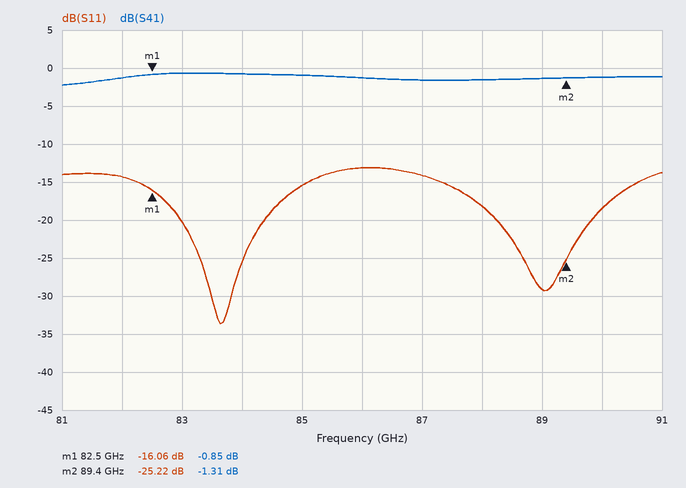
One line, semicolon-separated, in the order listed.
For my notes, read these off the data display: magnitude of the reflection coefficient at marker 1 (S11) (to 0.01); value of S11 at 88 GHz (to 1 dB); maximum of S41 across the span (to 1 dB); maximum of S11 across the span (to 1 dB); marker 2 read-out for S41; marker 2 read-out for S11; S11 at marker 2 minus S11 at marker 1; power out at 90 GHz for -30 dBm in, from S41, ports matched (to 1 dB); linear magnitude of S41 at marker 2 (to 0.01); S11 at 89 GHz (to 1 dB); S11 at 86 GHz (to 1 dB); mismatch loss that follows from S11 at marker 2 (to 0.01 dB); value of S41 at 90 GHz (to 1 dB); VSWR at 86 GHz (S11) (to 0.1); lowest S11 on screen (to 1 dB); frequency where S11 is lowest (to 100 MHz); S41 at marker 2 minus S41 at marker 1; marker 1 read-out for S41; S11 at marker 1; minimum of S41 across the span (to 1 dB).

0.16; -18 dB; -1 dB; -13 dB; -1.31 dB; -25.22 dB; -9.16 dB; -31 dBm; 0.86; -29 dB; -13 dB; 0.01 dB; -1 dB; 1.6; -34 dB; 83.6 GHz; -0.46 dB; -0.85 dB; -16.06 dB; -2 dB
